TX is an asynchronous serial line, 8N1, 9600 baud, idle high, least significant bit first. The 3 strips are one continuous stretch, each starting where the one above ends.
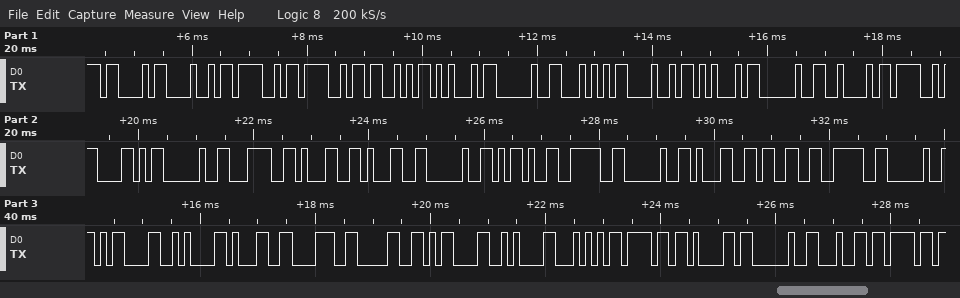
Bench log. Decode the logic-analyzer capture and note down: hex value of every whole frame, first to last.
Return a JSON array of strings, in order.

["43 48 4F 4F 53 45 20 54 48 45 20 42 4F 58 20 3C 31 31 20 2D 3E 20 31 33 3E 20 0D 0A 31 38 30 0D 0A 54 6F 61 20 64 6F"]
